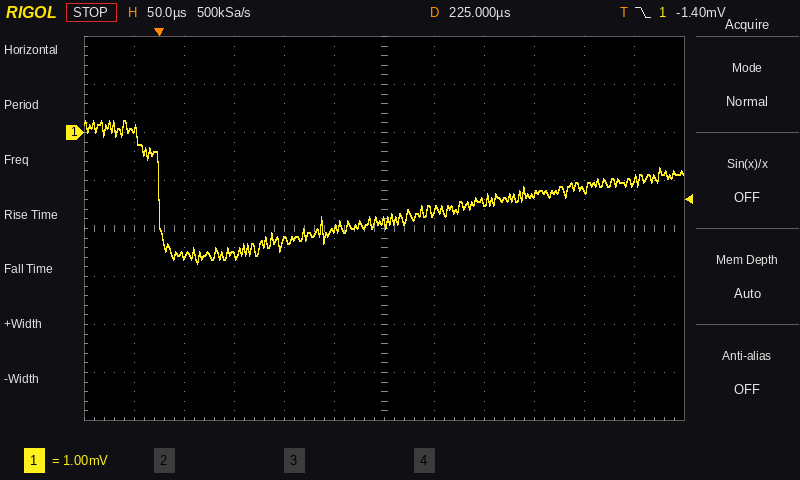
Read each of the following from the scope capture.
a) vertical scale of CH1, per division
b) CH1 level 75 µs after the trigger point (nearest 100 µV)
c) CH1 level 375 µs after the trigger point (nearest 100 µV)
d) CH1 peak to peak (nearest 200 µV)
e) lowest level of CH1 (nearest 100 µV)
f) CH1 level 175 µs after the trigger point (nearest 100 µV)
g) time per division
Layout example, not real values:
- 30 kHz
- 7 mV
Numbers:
- 1 mV
- -2.6 mV
- -1.3 mV
- 3.0 mV
- -2.7 mV
- -2.0 mV
- 50 µs
